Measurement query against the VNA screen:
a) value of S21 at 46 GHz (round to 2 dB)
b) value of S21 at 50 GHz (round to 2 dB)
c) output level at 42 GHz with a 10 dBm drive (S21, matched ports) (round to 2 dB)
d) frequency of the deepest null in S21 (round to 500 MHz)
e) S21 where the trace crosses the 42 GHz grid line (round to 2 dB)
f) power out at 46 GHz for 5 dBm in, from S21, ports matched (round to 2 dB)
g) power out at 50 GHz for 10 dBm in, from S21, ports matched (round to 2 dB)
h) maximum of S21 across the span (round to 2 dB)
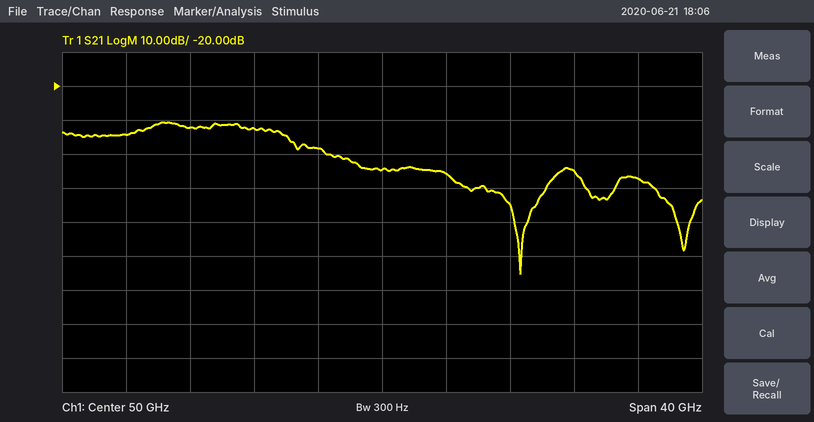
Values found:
-38 dB
-44 dB
-22 dBm
58.5 GHz
-32 dB
-34 dBm
-34 dBm
-30 dB
